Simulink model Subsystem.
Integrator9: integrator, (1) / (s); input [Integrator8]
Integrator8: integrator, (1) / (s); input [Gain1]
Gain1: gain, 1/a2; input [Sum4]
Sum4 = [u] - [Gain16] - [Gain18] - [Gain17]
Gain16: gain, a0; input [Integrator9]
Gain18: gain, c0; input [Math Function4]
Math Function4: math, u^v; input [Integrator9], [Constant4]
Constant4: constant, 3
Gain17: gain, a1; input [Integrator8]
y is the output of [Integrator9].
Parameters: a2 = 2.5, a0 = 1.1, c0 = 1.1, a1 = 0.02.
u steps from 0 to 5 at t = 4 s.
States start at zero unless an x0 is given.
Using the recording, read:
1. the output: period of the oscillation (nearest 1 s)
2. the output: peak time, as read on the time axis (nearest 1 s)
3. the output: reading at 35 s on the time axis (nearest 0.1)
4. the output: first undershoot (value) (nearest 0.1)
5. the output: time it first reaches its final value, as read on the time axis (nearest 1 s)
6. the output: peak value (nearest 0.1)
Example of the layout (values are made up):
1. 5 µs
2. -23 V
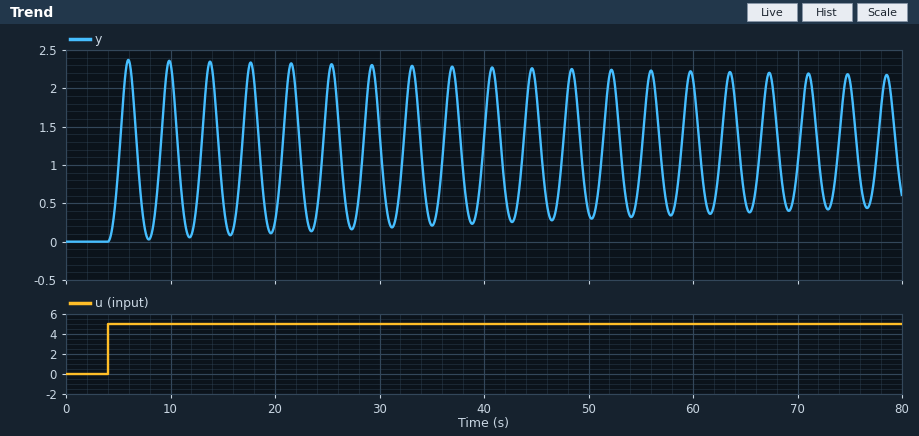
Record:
1. 4 s
2. 6 s
3. 0.2
4. 0.0
5. 5 s
6. 2.4
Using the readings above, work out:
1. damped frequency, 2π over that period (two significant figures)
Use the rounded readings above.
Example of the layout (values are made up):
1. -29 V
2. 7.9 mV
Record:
1. 1.6 rad/s
